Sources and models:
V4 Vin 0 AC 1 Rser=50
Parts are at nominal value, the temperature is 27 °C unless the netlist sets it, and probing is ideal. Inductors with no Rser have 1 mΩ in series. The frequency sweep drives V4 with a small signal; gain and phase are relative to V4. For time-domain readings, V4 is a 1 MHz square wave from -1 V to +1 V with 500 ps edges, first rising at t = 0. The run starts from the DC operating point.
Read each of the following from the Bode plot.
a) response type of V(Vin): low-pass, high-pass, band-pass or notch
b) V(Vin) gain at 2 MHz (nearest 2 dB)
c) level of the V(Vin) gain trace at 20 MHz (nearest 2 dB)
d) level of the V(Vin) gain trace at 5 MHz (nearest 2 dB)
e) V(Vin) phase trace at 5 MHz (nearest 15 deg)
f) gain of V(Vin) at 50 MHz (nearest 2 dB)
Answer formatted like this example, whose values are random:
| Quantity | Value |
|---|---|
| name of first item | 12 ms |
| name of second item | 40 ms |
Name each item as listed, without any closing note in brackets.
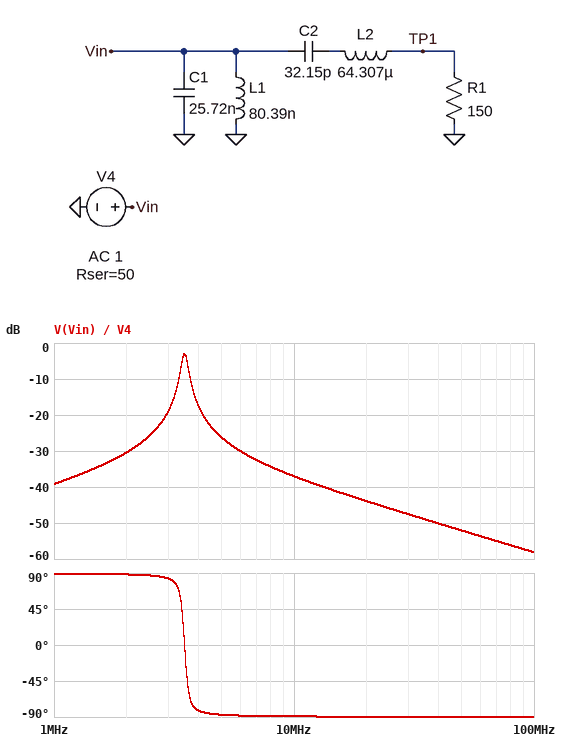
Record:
| Quantity | Value |
|---|---|
| response type of V(Vin): low-pass, high-pass, band-pass or notch | band-pass |
| V(Vin) gain at 2 MHz | -30 dB |
| level of the V(Vin) gain trace at 20 MHz | -44 dB |
| level of the V(Vin) gain trace at 5 MHz | -26 dB |
| V(Vin) phase trace at 5 MHz | -90 deg |
| gain of V(Vin) at 50 MHz | -52 dB |
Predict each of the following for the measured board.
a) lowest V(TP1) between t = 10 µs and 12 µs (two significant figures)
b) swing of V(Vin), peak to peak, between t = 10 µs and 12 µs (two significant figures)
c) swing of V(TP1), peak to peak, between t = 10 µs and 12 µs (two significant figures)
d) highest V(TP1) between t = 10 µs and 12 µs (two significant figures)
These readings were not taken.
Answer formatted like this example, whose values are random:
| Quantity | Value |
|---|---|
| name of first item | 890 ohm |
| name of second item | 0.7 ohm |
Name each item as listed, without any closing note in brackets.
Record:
| Quantity | Value |
|---|---|
| lowest V(TP1) between t = 10 µs and 12 µs | -18 mV |
| swing of V(Vin), peak to peak, between t = 10 µs and 12 µs | 110 mV |
| swing of V(TP1), peak to peak, between t = 10 µs and 12 µs | 36 mV |
| highest V(TP1) between t = 10 µs and 12 µs | 18 mV |
